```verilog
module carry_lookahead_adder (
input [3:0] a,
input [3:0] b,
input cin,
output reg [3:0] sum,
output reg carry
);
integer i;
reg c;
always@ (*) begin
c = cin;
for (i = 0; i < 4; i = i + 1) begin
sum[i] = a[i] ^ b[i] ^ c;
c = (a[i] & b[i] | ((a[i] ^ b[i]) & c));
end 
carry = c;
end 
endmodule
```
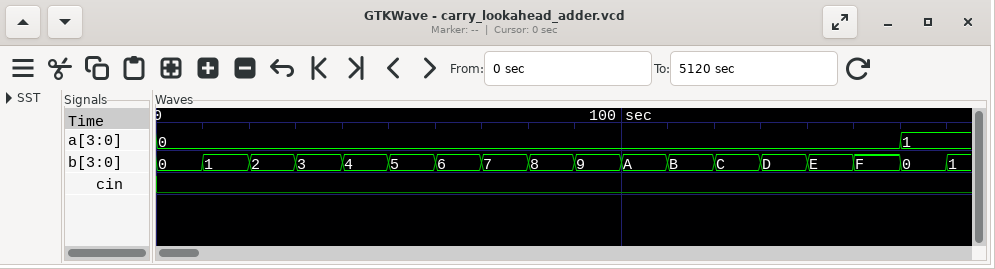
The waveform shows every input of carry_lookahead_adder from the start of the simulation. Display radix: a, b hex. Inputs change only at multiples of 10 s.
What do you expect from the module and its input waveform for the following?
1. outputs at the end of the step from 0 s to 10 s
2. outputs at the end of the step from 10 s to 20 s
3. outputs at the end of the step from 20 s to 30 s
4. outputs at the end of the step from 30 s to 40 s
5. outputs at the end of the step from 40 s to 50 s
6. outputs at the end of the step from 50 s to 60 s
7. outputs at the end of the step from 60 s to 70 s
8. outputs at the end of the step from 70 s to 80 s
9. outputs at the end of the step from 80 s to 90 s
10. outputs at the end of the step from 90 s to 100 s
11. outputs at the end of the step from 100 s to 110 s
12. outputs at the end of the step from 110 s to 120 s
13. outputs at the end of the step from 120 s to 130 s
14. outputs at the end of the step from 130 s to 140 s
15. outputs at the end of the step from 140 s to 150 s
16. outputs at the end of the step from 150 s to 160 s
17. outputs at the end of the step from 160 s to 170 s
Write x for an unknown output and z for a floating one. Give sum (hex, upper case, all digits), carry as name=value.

sum=0, carry=0
sum=1, carry=0
sum=2, carry=0
sum=3, carry=0
sum=4, carry=0
sum=5, carry=0
sum=6, carry=0
sum=7, carry=0
sum=8, carry=0
sum=9, carry=0
sum=A, carry=0
sum=B, carry=0
sum=C, carry=0
sum=D, carry=0
sum=E, carry=0
sum=F, carry=0
sum=1, carry=0
